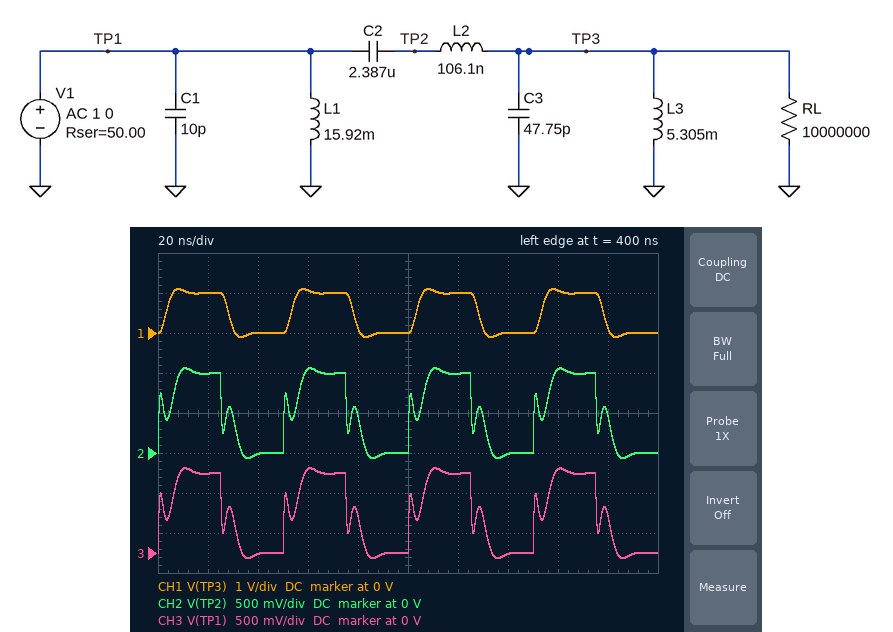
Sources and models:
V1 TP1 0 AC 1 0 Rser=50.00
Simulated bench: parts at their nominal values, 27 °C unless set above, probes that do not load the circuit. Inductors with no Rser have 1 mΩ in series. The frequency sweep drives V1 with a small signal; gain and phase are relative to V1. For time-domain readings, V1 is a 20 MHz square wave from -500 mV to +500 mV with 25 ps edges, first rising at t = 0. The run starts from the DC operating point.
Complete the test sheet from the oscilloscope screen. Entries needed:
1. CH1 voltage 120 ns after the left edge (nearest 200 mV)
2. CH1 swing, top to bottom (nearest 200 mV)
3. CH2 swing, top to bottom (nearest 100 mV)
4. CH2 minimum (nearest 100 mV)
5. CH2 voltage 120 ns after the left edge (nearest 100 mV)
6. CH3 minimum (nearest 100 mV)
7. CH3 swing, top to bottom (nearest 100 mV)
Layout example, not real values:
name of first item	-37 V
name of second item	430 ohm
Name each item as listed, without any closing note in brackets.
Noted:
CH1 voltage 120 ns after the left edge	1.0 V
CH1 swing, top to bottom	1.2 V
CH2 swing, top to bottom	1.1 V
CH2 minimum	-100 mV
CH2 voltage 120 ns after the left edge	1.0 V
CH3 minimum	-100 mV
CH3 swing, top to bottom	1.1 V
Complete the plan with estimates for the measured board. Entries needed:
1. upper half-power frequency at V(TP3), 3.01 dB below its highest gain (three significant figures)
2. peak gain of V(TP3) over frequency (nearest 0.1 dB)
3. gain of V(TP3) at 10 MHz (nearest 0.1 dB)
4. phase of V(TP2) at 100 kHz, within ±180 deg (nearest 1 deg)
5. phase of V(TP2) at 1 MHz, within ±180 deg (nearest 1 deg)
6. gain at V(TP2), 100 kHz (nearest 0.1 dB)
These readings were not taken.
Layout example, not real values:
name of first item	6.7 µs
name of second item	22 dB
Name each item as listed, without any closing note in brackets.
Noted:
upper half-power frequency at V(TP3), 3.01 dB below its highest gain	91.8 MHz
peak gain of V(TP3) over frequency	0.3 dB
gain of V(TP3) at 10 MHz	0 dB
phase of V(TP2) at 100 kHz, within ±180 deg	1 deg
phase of V(TP2) at 1 MHz, within ±180 deg	-1 deg
gain at V(TP2), 100 kHz	0 dB
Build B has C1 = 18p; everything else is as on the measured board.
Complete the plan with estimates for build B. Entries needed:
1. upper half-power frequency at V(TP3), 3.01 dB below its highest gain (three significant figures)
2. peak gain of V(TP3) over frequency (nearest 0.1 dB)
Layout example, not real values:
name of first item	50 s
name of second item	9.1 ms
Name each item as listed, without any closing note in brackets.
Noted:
upper half-power frequency at V(TP3), 3.01 dB below its highest gain	102 MHz
peak gain of V(TP3) over frequency	0 dB
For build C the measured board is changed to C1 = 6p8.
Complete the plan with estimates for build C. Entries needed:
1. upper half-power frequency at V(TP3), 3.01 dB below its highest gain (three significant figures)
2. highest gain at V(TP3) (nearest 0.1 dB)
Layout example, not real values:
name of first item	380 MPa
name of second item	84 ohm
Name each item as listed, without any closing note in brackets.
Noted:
upper half-power frequency at V(TP3), 3.01 dB below its highest gain	88.0 MHz
highest gain at V(TP3)	0.5 dB
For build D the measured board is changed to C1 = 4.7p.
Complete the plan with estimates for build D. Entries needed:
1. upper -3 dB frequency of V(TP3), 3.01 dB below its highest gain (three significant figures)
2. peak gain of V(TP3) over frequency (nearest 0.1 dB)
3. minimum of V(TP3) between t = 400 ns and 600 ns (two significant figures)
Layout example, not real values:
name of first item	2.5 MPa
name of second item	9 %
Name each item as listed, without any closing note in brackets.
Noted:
upper -3 dB frequency of V(TP3), 3.01 dB below its highest gain	85.8 MHz
peak gain of V(TP3) over frequency	0.6 dB
minimum of V(TP3) between t = 400 ns and 600 ns	-120 mV
